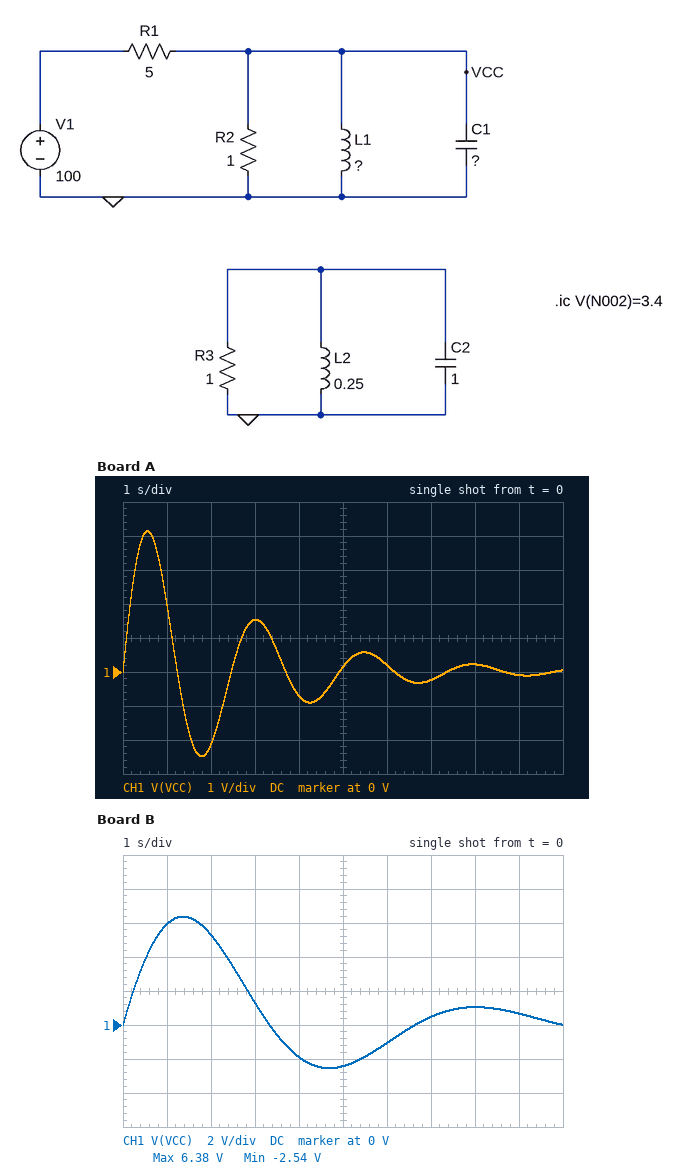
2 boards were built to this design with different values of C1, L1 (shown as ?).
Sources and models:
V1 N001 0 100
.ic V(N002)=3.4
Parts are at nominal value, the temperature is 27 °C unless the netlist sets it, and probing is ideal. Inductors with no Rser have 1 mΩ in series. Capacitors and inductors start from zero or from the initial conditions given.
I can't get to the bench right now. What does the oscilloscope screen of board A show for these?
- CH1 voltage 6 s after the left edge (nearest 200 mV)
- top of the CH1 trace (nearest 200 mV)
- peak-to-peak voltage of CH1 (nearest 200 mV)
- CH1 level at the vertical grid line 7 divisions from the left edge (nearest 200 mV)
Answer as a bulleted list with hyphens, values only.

- 200 mV
- 4.2 V
- 6.6 V
- -200 mV
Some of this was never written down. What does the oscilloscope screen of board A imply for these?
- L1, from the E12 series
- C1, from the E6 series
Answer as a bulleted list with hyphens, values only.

- 100 mH
- 1.5 F
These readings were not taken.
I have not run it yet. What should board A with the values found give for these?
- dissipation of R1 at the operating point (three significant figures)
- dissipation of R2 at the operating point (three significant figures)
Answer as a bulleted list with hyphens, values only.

- 2.00 kW
- 399 µW
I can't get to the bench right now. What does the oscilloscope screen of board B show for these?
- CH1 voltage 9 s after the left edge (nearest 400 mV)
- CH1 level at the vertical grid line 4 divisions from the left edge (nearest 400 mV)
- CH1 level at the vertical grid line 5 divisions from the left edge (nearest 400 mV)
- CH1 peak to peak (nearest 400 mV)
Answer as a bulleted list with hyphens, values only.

- 800 mV
- -2.0 V
- -2.4 V
- 8.8 V
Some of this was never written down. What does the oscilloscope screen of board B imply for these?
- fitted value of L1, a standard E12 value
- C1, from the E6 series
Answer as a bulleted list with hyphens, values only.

- 470 mH
- 2.2 F
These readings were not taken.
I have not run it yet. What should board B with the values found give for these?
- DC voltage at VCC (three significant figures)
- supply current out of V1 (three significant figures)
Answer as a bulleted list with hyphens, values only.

- 20.0 mV
- 20.0 A
